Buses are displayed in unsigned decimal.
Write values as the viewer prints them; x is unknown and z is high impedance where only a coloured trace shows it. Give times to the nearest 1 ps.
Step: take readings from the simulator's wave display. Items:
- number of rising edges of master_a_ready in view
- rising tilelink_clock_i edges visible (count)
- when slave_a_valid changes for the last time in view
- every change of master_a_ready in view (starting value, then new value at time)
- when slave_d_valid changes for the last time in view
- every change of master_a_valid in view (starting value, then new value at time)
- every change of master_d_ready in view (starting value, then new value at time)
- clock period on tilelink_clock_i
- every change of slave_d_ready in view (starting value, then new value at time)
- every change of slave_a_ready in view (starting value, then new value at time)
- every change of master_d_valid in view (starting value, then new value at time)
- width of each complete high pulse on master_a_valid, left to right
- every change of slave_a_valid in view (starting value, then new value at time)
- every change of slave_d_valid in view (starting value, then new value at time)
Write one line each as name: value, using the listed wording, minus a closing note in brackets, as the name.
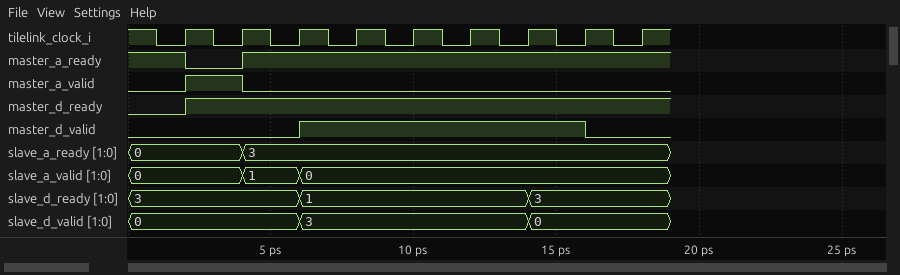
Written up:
number of rising edges of master_a_ready in view: 1
rising tilelink_clock_i edges visible: 9
when slave_a_valid changes for the last time in view: 6 ps
every change of master_a_ready in view: 1, 0 at 2 ps, 1 at 4 ps
when slave_d_valid changes for the last time in view: 14 ps
every change of master_a_valid in view: 0, 1 at 2 ps, 0 at 4 ps
every change of master_d_ready in view: 0, 1 at 2 ps
clock period on tilelink_clock_i: 2 ps
every change of slave_d_ready in view: 3, 1 at 6 ps, 3 at 14 ps
every change of slave_a_ready in view: 0, 3 at 4 ps
every change of master_d_valid in view: 0, 1 at 6 ps, 0 at 16 ps
width of each complete high pulse on master_a_valid, left to right: 2 ps
every change of slave_a_valid in view: 0, 1 at 4 ps, 0 at 6 ps
every change of slave_d_valid in view: 0, 3 at 6 ps, 0 at 14 ps
